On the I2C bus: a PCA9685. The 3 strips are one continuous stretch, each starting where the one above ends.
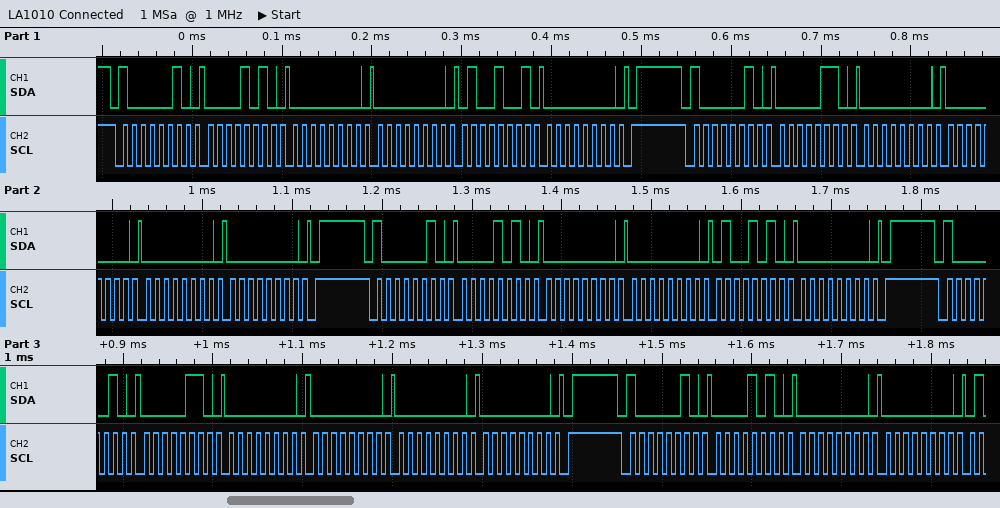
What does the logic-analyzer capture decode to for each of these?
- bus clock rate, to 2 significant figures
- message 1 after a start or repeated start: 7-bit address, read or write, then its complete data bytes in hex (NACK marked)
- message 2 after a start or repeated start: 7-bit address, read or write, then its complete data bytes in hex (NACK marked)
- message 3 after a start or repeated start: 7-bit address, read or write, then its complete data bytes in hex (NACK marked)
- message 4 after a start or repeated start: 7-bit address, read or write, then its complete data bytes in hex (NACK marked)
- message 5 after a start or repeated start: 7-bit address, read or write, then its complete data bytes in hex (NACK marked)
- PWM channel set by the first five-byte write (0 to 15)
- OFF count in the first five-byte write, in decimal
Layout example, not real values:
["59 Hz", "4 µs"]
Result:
["100 kHz", "0x41 write: 0A 00 00 49 00", "0x41 write: 06 00 00 00 00", "0x41 write: 0A 00 00 4A 00", "0x41 write: 06 00 00 00 00", "0x41 write: 0A 00 00", "1", "73"]
